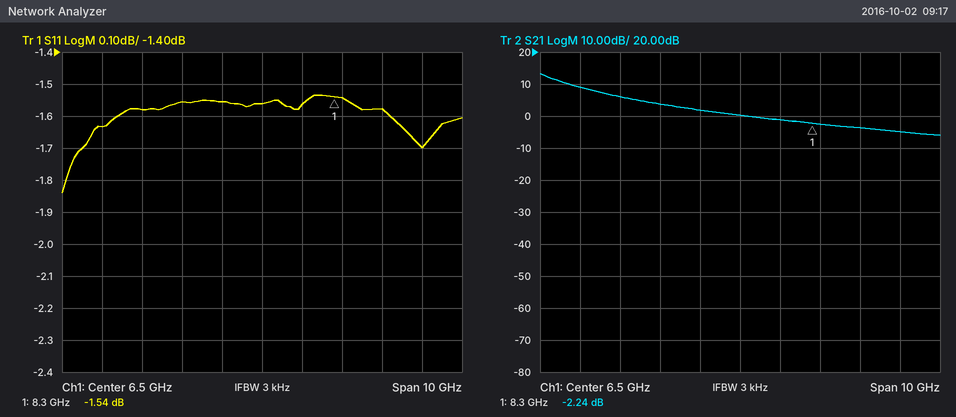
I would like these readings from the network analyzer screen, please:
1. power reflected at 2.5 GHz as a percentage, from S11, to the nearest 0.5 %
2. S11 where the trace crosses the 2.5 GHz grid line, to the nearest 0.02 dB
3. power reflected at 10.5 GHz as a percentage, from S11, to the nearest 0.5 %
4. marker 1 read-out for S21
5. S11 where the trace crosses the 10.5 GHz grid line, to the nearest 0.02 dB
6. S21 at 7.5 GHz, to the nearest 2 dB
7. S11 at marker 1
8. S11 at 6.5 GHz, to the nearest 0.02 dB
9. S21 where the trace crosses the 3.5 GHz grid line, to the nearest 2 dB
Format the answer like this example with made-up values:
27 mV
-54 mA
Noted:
68.5 %
-1.64 dB
67.5 %
-2.24 dB
-1.70 dB
-2 dB
-1.54 dB
-1.56 dB
6 dB
